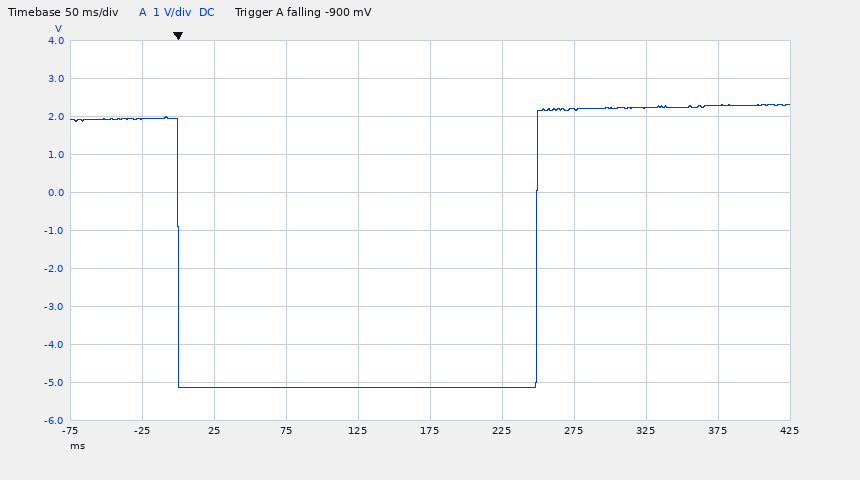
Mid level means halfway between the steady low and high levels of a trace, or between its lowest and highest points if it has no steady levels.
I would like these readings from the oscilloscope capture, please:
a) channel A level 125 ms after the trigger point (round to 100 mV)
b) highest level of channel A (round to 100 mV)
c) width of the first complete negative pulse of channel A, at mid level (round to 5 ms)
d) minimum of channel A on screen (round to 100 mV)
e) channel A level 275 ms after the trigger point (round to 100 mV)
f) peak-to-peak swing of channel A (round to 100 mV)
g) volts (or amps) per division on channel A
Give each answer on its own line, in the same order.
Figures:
-5.1 V
2.3 V
250 ms
-5.1 V
2.2 V
7.4 V
1 V
